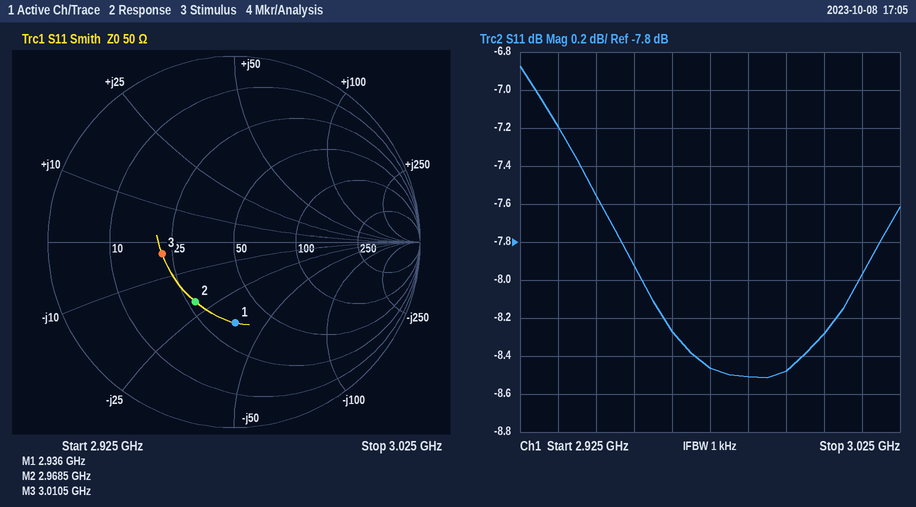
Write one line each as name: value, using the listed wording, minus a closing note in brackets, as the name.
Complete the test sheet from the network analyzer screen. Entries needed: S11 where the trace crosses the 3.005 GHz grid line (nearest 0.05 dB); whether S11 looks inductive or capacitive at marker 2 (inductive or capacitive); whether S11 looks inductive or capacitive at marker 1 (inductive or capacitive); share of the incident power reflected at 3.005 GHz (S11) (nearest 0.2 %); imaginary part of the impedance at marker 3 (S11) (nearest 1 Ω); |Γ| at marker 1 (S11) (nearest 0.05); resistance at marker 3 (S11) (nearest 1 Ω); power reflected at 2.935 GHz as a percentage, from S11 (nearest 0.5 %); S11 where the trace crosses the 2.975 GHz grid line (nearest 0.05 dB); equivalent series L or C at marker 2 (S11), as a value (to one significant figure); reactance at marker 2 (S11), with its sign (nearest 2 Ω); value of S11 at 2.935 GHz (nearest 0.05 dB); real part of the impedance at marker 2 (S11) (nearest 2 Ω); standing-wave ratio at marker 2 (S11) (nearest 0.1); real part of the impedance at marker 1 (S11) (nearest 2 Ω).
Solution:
S11 where the trace crosses the 3.005 GHz grid line: -8.30 dB
whether S11 looks inductive or capacitive at marker 2: capacitive
whether S11 looks inductive or capacitive at marker 1: capacitive
share of the incident power reflected at 3.005 GHz (S11): 14.8 %
imaginary part of the impedance at marker 3 (S11): -3 Ω
|Γ| at marker 1 (S11): 0.45
resistance at marker 3 (S11): 22 Ω
power reflected at 2.935 GHz as a percentage, from S11: 19.0 %
S11 where the trace crosses the 2.975 GHz grid line: -8.45 dB
equivalent series L or C at marker 2 (S11), as a value: 3 pF
reactance at marker 2 (S11), with its sign: -20 Ω
value of S11 at 2.935 GHz: -7.20 dB
real part of the impedance at marker 2 (S11): 28 Ω
standing-wave ratio at marker 2 (S11): 2.2
real part of the impedance at marker 1 (S11): 34 Ω
